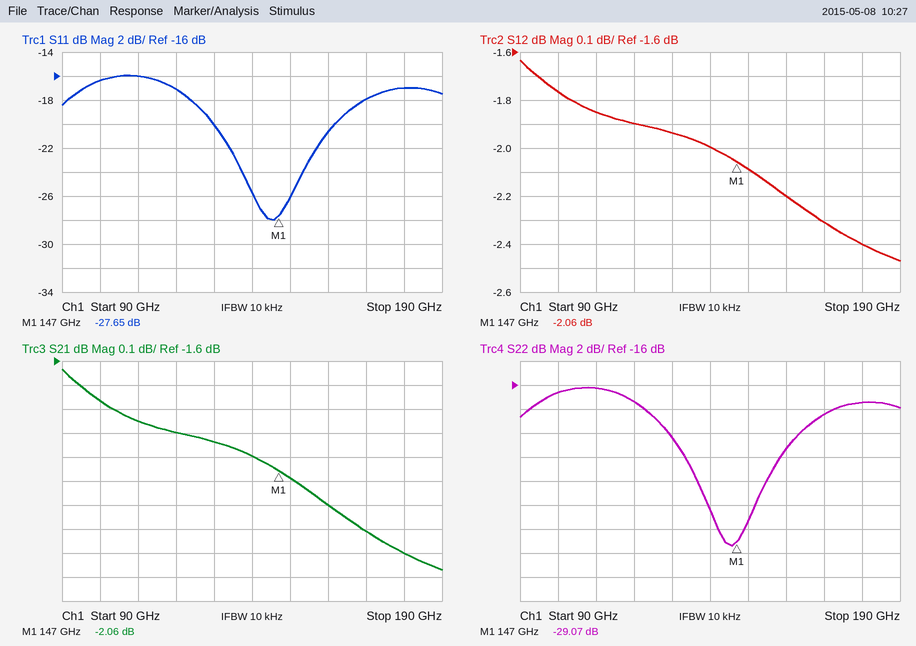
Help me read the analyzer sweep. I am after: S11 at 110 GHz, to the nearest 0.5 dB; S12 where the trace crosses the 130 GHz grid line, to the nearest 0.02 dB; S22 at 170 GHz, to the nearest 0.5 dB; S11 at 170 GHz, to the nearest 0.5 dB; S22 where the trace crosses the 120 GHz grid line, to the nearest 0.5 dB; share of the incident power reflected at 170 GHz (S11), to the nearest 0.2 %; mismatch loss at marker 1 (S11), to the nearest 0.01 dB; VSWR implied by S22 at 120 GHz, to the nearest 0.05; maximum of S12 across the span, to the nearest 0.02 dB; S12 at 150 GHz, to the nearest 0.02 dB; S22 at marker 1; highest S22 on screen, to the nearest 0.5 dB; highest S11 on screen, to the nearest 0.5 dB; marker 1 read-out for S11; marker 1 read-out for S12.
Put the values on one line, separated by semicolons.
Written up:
-16.0 dB; -1.94 dB; -18.5 dB; -18.0 dB; -17.5 dB; 1.6 %; 0.01 dB; 1.30; -1.64 dB; -2.08 dB; -29.07 dB; -16.0 dB; -16.0 dB; -27.65 dB; -2.06 dB
